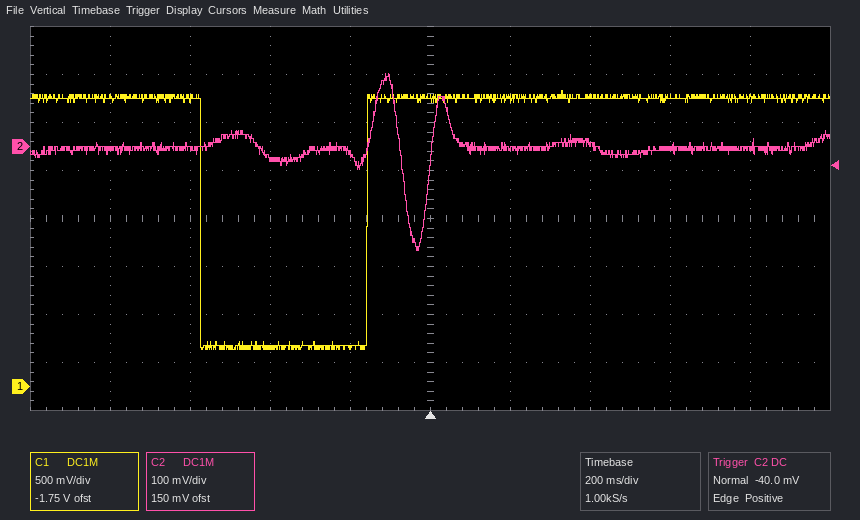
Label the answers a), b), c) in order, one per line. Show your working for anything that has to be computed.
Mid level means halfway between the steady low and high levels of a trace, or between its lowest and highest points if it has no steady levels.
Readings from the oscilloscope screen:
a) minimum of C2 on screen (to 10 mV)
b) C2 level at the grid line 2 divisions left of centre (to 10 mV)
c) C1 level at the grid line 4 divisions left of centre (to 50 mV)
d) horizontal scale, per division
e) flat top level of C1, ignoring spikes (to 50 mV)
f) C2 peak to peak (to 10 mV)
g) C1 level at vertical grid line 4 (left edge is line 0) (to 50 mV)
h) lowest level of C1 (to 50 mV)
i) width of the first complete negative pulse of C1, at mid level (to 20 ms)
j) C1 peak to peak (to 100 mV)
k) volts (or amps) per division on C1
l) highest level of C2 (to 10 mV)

a) -220 mV
b) -20 mV
c) 3.00 V
d) 200 ms
e) 3.00 V
f) 150 mV − (-220 mV) = 370 mV
g) 400 mV
h) 400 mV
i) 420 ms
j) 2.70 V
k) 500 mV
l) 150 mV
